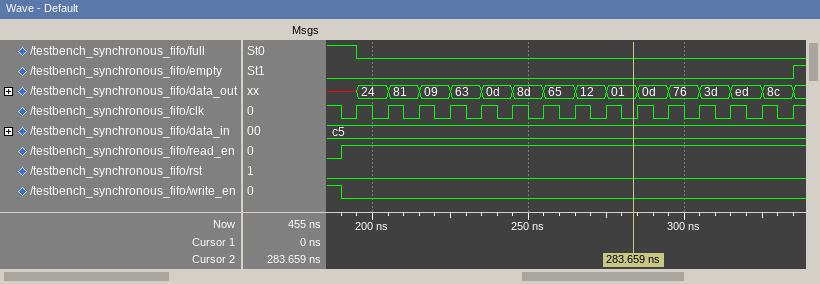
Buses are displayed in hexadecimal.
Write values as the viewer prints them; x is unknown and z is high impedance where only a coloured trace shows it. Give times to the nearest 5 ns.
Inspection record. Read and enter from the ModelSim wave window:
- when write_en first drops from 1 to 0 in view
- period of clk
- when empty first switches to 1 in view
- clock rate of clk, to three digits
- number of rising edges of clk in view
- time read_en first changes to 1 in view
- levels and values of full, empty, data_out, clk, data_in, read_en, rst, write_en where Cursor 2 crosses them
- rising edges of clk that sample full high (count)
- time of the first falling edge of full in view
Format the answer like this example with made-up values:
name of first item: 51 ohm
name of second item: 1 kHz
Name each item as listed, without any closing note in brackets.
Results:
when write_en first drops from 1 to 0 in view: 190 ns
period of clk: 10 ns
when empty first switches to 1 in view: 335 ns
clock rate of clk, to three digits: 100 MHz
number of rising edges of clk in view: 15
time read_en first changes to 1 in view: 190 ns
levels and values of full, empty, data_out, clk, data_in, read_en, rst, write_en where Cursor 2 crosses them: full=0, empty=0, data_out=01, clk=0, data_in=c5, read_en=1, rst=0, write_en=0
rising edges of clk that sample full high: 1
time of the first falling edge of full in view: 195 ns
